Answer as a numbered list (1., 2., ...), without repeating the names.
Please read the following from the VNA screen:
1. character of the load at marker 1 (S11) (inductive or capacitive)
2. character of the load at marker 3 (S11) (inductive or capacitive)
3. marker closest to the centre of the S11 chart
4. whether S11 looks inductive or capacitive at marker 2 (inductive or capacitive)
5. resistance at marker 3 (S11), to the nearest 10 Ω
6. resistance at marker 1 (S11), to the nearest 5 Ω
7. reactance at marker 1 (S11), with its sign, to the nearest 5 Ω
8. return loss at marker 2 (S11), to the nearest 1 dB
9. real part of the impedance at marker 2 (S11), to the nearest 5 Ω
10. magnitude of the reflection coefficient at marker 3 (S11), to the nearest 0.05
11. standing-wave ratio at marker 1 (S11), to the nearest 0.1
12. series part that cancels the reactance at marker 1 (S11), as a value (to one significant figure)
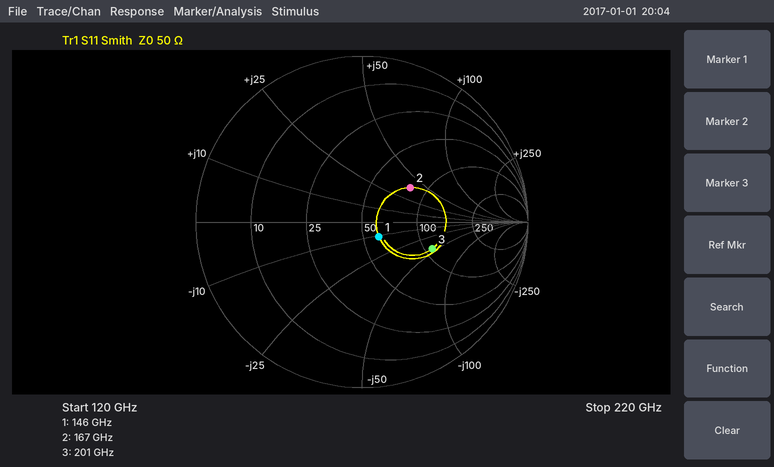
1. capacitive
2. capacitive
3. marker 1
4. inductive
5. 110 Ω
6. 60 Ω
7. -10 Ω
8. 9 dB
9. 80 Ω
10. 0.45
11. 1.3
12. 10 pH
